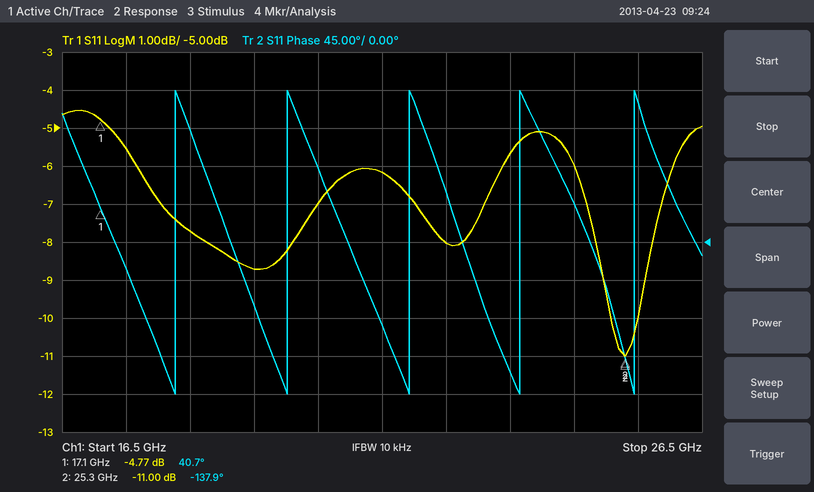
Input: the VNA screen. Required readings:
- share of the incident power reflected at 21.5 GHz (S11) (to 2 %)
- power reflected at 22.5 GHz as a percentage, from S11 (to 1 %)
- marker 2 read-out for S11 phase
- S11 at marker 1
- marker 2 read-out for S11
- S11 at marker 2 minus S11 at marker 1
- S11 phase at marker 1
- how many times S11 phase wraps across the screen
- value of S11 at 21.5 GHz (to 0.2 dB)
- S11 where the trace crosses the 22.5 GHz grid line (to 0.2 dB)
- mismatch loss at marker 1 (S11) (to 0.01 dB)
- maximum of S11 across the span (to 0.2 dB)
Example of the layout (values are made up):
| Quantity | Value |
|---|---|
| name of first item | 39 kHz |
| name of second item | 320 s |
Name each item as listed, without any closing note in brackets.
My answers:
| Quantity | Value |
|---|---|
| share of the incident power reflected at 21.5 GHz (S11) | 24 % |
| power reflected at 22.5 GHz as a percentage, from S11 | 16 % |
| marker 2 read-out for S11 phase | -137.9° |
| S11 at marker 1 | -4.77 dB |
| marker 2 read-out for S11 | -11.00 dB |
| S11 at marker 2 minus S11 at marker 1 | -6.23 dB |
| S11 phase at marker 1 | 40.7° |
| how many times S11 phase wraps across the screen | 5 |
| value of S11 at 21.5 GHz | -6.2 dB |
| S11 where the trace crosses the 22.5 GHz grid line | -8.0 dB |
| mismatch loss at marker 1 (S11) | 1.76 dB |
| maximum of S11 across the span | -4.6 dB |
